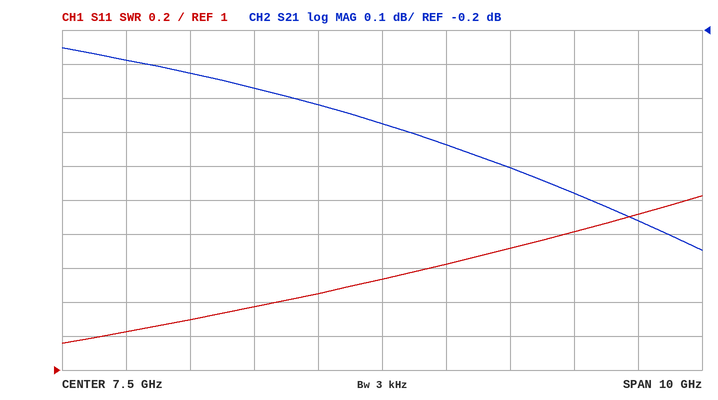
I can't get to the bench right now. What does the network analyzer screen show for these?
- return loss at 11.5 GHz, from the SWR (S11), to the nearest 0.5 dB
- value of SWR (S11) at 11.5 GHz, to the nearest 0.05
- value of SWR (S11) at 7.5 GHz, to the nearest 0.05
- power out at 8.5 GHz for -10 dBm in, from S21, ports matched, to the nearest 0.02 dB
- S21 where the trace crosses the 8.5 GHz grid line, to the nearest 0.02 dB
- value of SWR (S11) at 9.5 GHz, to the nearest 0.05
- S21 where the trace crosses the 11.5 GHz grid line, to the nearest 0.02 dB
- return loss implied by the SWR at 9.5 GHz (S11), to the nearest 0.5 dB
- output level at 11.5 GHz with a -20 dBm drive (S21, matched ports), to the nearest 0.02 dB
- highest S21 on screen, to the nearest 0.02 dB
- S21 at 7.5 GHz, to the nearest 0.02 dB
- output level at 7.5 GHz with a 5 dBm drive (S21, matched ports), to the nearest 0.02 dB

10.0 dB
1.90
1.55
-10.54 dBm
-0.54 dB
1.70
-0.76 dB
11.5 dB
-20.76 dBm
-0.26 dB
-0.48 dB
4.52 dBm
